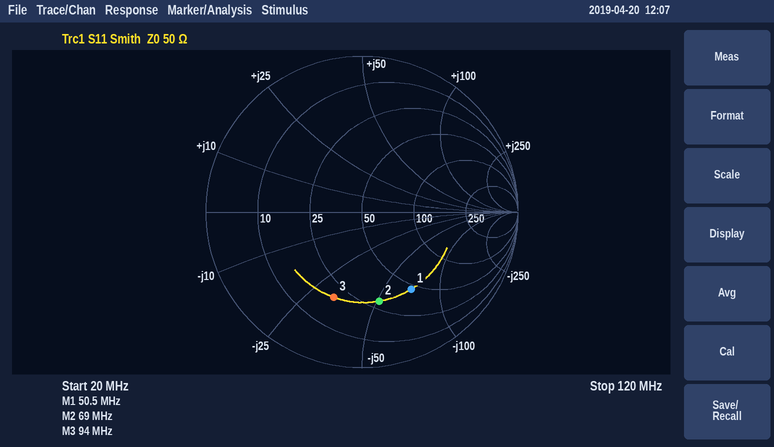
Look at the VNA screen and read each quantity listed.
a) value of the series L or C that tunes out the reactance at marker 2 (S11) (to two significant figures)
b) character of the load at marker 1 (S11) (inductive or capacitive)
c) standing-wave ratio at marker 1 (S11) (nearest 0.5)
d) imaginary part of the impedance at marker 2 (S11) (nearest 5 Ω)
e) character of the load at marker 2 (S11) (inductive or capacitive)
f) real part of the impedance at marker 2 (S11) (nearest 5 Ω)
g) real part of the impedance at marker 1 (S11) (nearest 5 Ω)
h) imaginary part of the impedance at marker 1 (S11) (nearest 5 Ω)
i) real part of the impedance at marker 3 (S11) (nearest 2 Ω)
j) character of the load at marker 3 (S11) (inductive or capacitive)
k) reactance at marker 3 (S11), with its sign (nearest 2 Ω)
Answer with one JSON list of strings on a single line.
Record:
["120 nH", "capacitive", "4.0", "-50 Ω", "capacitive", "30 Ω", "45 Ω", "-70 Ω", "20 Ω", "capacitive", "-32 Ω"]
